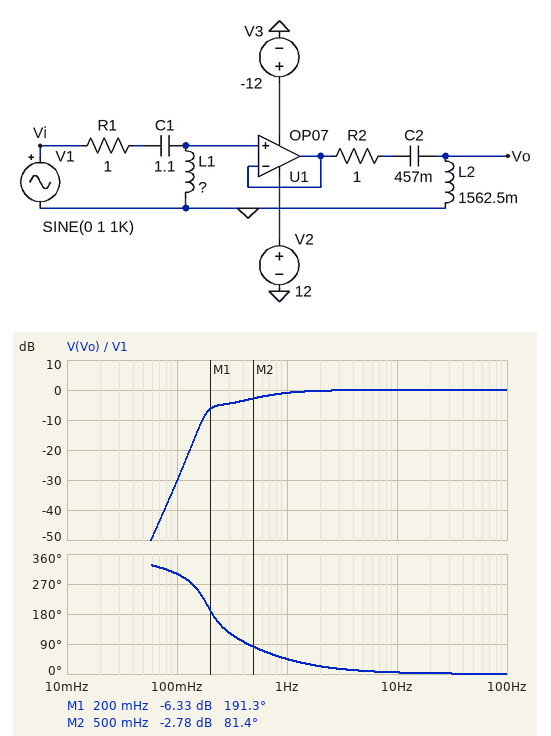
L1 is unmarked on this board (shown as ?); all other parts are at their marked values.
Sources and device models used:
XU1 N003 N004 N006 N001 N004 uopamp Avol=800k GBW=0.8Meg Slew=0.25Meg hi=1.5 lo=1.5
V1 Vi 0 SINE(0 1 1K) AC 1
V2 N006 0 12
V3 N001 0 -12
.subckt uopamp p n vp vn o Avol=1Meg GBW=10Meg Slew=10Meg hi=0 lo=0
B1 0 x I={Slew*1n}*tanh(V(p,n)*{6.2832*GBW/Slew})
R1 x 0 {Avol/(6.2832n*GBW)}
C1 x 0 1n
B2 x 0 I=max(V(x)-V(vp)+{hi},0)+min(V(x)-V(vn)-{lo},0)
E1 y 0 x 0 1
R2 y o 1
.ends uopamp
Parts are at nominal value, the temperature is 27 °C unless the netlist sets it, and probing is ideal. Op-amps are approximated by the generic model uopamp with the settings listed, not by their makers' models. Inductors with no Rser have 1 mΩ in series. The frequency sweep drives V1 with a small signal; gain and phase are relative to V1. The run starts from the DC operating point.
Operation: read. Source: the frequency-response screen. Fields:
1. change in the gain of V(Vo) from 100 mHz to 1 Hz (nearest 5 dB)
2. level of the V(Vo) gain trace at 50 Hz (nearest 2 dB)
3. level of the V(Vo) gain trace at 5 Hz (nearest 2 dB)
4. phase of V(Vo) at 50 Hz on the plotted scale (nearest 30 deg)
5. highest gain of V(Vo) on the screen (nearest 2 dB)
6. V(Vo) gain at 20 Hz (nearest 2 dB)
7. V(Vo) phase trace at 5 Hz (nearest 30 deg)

30 dB
0 dB
0 dB
0 deg
0 dB
0 dB
0 deg
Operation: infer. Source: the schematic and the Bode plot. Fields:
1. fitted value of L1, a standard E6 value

220 mH
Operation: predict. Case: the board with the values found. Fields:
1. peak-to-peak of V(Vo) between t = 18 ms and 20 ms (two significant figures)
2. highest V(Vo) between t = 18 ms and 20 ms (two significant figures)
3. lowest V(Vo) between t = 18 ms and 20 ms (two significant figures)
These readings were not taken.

2.0 V
1.0 V
-1.0 V
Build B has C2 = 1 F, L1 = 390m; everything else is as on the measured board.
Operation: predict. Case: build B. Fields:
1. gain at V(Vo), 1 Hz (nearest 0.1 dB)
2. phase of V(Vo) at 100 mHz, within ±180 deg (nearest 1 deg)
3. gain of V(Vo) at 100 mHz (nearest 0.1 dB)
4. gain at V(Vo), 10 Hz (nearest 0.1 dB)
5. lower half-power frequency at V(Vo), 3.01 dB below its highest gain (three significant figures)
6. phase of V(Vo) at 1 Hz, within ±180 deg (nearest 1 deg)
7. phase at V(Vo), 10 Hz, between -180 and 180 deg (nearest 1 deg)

-0.1 dB
-99 deg
-17.6 dB
0 dB
242 mHz
29 deg
3 deg
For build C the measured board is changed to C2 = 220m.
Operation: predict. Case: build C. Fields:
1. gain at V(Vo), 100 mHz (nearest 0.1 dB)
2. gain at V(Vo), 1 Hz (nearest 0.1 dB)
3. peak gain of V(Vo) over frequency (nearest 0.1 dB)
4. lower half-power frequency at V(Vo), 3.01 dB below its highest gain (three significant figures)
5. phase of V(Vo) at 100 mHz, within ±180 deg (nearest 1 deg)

-37.7 dB
-0.6 dB
0.6 dB
250 mHz
-47 deg
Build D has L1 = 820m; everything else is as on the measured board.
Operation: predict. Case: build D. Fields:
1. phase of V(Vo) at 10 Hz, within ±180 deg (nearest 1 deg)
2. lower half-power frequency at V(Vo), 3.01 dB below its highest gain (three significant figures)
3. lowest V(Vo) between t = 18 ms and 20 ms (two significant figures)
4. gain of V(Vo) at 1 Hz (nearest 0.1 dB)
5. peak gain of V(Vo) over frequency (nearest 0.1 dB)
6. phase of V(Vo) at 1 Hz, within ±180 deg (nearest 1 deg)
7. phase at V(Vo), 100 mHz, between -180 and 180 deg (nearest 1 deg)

2 deg
170 mHz
-1.0 V
0.3 dB
5.7 dB
17 deg
-69 deg
